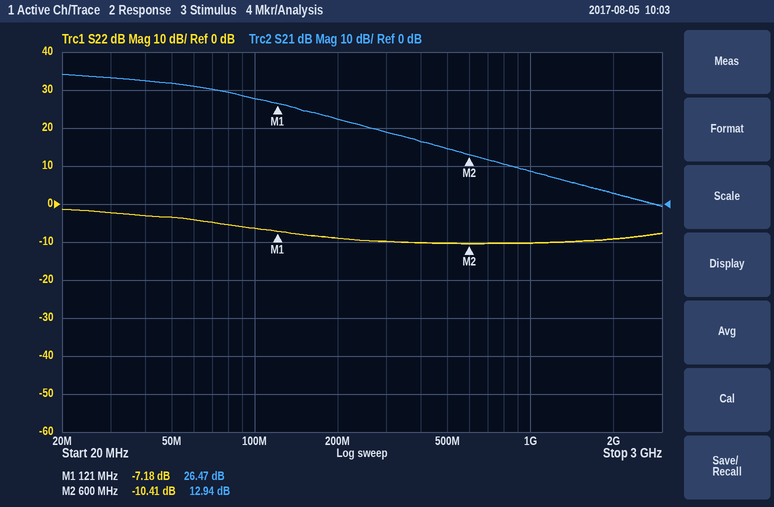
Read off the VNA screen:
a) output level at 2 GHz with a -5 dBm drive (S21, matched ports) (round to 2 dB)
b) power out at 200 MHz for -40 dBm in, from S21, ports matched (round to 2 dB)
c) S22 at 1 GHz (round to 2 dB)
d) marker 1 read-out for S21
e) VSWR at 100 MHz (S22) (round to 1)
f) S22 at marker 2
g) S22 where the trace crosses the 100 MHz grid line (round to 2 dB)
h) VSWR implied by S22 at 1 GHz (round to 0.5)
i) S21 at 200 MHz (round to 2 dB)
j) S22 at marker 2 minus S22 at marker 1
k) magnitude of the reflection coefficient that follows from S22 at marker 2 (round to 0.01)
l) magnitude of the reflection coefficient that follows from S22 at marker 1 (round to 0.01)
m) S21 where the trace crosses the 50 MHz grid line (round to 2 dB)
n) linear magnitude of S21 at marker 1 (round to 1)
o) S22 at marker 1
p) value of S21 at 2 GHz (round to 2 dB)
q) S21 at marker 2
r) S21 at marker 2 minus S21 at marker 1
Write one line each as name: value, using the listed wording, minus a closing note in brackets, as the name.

output level at 2 GHz with a -5 dBm drive (S21, matched ports): -2 dBm
power out at 200 MHz for -40 dBm in, from S21, ports matched: -18 dBm
S22 at 1 GHz: -10 dB
marker 1 read-out for S21: 26.47 dB
VSWR at 100 MHz (S22): 3
S22 at marker 2: -10.41 dB
S22 where the trace crosses the 100 MHz grid line: -6 dB
VSWR implied by S22 at 1 GHz: 2.0
S21 at 200 MHz: 22 dB
S22 at marker 2 minus S22 at marker 1: -3.23 dB
magnitude of the reflection coefficient that follows from S22 at marker 2: 0.30
magnitude of the reflection coefficient that follows from S22 at marker 1: 0.44
S21 where the trace crosses the 50 MHz grid line: 32 dB
linear magnitude of S21 at marker 1: 21
S22 at marker 1: -7.18 dB
value of S21 at 2 GHz: 2 dB
S21 at marker 2: 12.94 dB
S21 at marker 2 minus S21 at marker 1: -13.53 dB
